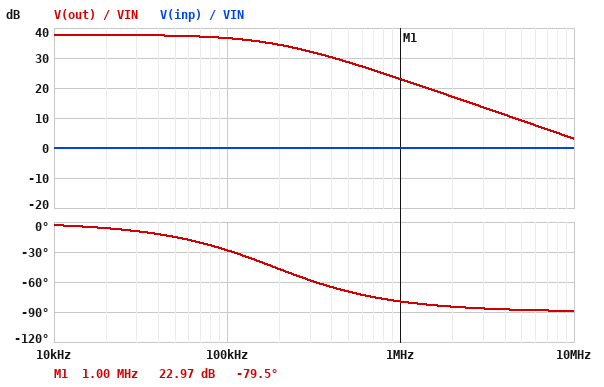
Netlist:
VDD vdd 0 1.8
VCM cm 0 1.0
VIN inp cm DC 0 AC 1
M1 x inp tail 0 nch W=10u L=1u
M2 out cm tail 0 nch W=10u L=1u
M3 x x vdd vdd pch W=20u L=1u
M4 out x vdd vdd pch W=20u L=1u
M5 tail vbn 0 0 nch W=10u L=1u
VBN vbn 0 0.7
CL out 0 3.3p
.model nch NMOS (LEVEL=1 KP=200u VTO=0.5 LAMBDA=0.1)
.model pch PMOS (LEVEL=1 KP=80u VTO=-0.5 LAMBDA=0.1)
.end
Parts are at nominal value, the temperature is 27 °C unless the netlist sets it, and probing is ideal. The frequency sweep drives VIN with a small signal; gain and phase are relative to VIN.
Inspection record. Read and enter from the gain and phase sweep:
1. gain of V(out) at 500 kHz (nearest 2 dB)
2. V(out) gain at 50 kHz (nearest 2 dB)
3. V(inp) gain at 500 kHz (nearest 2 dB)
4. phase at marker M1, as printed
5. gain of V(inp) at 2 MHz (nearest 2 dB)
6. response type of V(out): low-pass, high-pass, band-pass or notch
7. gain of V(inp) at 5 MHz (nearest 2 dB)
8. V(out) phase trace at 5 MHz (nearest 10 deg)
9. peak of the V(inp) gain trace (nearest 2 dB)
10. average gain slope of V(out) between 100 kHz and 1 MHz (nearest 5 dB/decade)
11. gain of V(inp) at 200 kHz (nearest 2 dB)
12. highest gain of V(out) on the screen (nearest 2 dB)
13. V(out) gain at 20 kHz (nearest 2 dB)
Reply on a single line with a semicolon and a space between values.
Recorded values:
28 dB; 38 dB; 0 dB; -79.5 deg; 0 dB; low-pass; 0 dB; -90 deg; 0 dB; -15 dB/decade; 0 dB; 38 dB; 38 dB
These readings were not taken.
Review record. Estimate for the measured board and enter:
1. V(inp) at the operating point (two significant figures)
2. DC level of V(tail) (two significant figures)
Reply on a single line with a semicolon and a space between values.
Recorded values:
1.0 V; 360 mV
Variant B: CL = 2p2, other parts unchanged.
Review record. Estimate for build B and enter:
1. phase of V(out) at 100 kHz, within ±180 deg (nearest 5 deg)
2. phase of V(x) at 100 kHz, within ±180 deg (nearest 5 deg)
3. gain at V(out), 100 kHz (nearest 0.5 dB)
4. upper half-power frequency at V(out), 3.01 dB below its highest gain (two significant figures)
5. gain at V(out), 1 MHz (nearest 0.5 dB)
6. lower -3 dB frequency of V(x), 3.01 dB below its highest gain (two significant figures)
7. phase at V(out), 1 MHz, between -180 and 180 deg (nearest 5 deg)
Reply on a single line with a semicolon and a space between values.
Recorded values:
-20 deg; -165 deg; 37.0 dB; 280 kHz; 26.5 dB; 190 kHz; -75 deg
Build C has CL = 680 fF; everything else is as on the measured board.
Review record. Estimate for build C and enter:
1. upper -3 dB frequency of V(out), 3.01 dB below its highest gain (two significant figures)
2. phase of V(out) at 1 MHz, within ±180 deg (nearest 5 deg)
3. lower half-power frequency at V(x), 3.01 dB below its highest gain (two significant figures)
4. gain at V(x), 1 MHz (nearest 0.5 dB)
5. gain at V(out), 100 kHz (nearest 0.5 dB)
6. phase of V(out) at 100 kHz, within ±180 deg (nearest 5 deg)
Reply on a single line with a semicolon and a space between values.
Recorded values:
900 kHz; -50 deg; 620 kHz; -7.0 dB; 37.5 dB; -5 deg
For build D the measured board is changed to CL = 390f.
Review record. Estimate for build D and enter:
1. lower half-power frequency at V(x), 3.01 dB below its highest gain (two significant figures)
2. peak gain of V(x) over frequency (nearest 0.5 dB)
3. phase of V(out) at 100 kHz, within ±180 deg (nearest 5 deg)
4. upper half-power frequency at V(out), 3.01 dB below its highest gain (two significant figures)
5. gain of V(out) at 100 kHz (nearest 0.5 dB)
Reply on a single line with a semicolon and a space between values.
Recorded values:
1.1 MHz; -5.0 dB; -5 deg; 1.6 MHz; 37.5 dB
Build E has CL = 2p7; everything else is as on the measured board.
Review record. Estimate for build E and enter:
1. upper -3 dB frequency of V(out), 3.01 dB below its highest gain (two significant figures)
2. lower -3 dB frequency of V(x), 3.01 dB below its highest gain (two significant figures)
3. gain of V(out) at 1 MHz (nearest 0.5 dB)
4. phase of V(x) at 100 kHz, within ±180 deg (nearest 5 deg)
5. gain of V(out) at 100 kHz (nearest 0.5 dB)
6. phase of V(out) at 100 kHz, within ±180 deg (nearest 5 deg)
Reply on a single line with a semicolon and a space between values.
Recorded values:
230 kHz; 160 kHz; 24.5 dB; -165 deg; 37.0 dB; -25 deg
